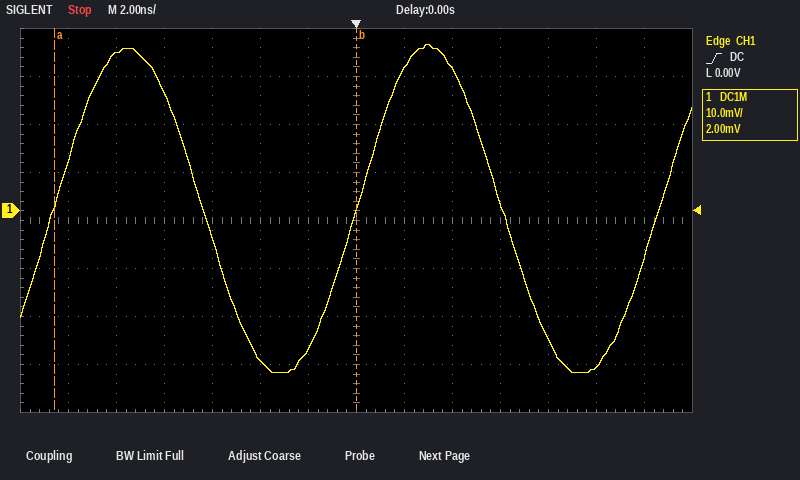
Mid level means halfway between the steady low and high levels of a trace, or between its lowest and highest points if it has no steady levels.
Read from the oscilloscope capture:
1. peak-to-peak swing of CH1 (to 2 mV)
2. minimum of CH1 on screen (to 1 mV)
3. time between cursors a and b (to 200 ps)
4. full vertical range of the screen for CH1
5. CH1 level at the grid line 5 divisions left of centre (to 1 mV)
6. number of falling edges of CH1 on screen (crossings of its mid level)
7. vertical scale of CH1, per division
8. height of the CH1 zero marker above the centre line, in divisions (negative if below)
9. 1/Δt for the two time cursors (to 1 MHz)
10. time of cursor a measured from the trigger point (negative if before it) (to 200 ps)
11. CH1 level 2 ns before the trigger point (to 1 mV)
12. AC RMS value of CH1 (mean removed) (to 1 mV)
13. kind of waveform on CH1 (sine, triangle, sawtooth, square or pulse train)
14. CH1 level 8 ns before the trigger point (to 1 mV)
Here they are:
68 mV
-34 mV
12.6 ns
80 mV
33 mV
2
10 mV
+0.2 div
79 MHz
-12.6 ns
-29 mV
24 mV
sine
25 mV
